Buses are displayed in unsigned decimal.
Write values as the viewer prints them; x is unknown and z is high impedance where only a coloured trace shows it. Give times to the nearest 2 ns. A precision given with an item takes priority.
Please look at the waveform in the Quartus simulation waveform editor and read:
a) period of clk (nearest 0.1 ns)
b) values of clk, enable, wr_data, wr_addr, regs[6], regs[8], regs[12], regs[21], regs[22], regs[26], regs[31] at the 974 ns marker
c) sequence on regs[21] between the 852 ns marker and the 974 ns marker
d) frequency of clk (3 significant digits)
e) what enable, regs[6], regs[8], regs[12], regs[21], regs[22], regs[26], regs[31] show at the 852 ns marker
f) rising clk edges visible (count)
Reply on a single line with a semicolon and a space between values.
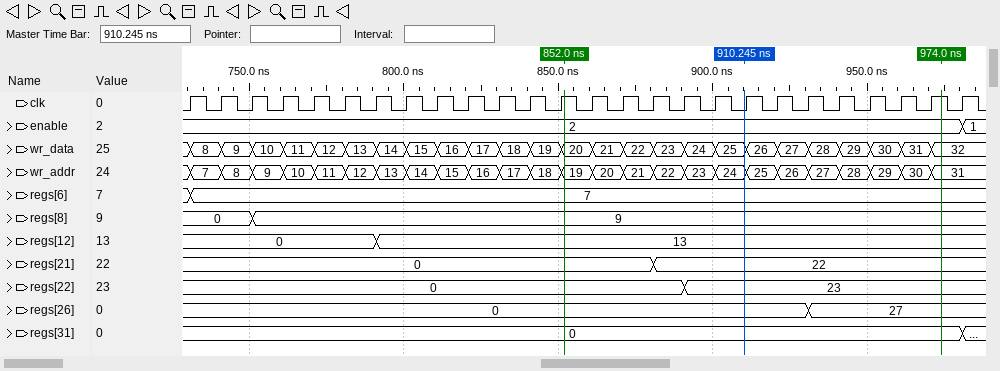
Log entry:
10 ns; clk=1, enable=2, wr_data=32, wr_addr=31, regs[6]=7, regs[8]=9, regs[12]=13, regs[21]=22, regs[22]=23, regs[26]=27, regs[31]=0; 0, 22; 100 MHz; enable=2, regs[6]=7, regs[8]=9, regs[12]=13, regs[21]=0, regs[22]=0, regs[26]=0, regs[31]=0; 26
